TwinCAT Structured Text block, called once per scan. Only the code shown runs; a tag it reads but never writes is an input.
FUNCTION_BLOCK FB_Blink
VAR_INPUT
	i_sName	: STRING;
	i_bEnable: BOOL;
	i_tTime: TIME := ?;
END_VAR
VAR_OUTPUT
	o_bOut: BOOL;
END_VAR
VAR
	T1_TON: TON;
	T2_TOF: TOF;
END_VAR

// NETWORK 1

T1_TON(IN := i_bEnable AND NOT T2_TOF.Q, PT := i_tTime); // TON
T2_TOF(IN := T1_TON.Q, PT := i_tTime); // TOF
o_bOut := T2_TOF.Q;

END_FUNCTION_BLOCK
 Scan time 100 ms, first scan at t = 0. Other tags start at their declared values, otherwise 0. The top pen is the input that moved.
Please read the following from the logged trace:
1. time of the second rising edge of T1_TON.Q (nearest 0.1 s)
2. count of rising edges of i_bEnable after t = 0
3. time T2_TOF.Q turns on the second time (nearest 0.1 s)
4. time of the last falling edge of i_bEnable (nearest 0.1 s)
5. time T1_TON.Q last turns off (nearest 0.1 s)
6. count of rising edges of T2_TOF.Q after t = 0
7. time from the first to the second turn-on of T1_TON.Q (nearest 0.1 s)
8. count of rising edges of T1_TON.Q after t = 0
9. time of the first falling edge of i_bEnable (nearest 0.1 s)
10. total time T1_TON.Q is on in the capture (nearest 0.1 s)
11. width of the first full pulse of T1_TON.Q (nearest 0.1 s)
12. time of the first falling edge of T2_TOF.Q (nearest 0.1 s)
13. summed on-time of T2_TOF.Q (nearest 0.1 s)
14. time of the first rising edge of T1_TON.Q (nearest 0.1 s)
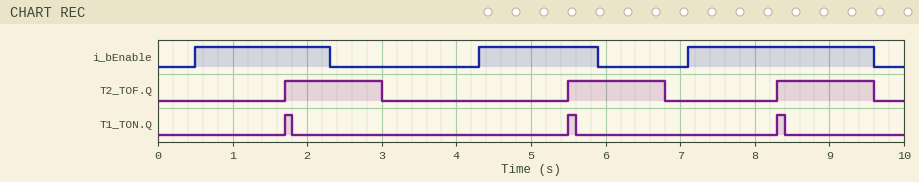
5.5 s
3
5.5 s
9.6 s
8.4 s
3
3.8 s
3
2.3 s
0.3 s
0.1 s
3.0 s
3.9 s
1.7 s
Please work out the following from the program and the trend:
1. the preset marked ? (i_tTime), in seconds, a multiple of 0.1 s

1.2 s
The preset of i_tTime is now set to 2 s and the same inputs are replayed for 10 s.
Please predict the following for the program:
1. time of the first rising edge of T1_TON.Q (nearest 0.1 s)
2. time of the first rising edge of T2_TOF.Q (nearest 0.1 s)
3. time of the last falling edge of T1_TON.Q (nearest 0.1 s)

9.1 s
9.1 s
9.2 s
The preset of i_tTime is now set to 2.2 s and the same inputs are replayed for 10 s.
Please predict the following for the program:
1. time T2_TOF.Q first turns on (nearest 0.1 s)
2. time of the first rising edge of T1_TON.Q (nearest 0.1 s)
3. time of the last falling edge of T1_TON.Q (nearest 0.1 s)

9.3 s
9.3 s
9.4 s
